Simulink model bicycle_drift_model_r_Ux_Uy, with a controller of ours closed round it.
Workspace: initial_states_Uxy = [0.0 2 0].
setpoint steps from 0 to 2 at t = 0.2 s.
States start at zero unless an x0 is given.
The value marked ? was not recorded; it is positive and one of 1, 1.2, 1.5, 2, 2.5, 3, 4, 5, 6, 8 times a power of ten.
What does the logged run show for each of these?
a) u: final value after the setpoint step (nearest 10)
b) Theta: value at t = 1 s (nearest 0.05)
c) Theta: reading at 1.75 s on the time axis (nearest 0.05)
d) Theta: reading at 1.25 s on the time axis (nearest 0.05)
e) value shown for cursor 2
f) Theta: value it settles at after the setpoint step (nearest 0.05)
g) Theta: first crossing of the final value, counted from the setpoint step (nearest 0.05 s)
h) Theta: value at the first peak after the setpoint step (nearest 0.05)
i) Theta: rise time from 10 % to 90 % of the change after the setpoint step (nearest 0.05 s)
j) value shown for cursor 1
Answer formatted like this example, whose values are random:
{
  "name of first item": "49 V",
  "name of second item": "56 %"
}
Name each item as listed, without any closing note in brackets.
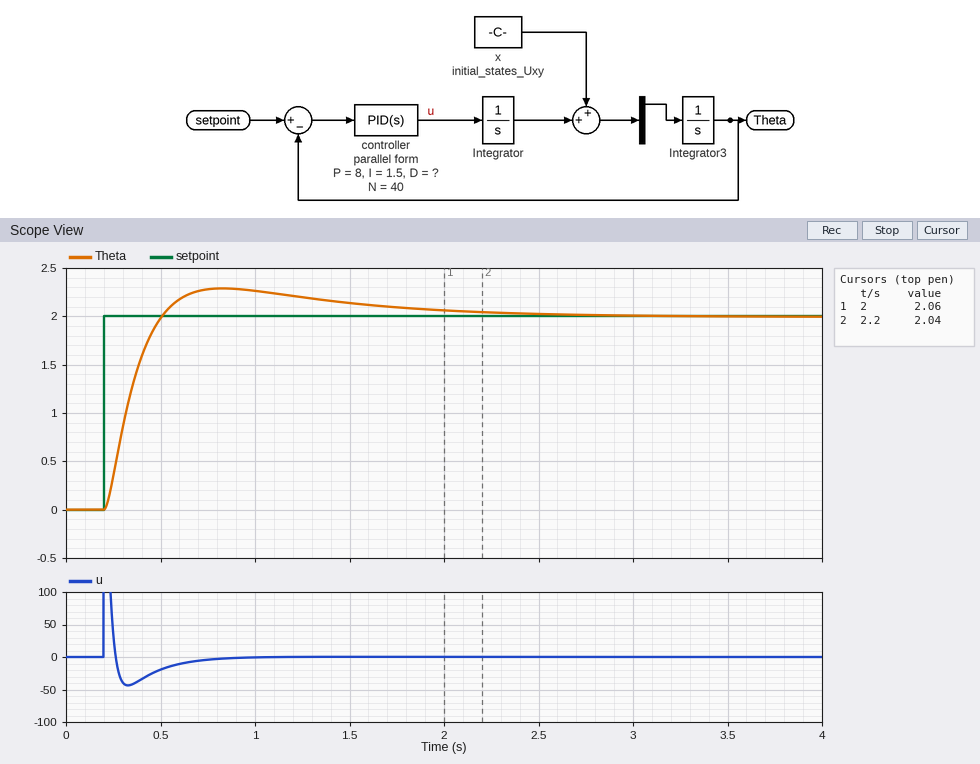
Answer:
{
  "u: final value after the setpoint step": "0",
  "Theta: value at t = 1 s": "2.25",
  "Theta: reading at 1.75 s on the time axis": "2.10",
  "Theta: reading at 1.25 s on the time axis": "2.20",
  "value shown for cursor 2": "2.04",
  "Theta: value it settles at after the setpoint step": "2.00",
  "Theta: first crossing of the final value, counted from the setpoint step": "0.30 s",
  "Theta: value at the first peak after the setpoint step": "2.30",
  "Theta: rise time from 10 % to 90 % of the change after the setpoint step": "0.20 s",
  "value shown for cursor 1": "2.06"
}
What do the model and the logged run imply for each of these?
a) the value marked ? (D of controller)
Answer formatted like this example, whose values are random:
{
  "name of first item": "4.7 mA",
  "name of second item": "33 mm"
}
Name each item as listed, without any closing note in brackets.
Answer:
{
  "the value marked ?": "6"
}
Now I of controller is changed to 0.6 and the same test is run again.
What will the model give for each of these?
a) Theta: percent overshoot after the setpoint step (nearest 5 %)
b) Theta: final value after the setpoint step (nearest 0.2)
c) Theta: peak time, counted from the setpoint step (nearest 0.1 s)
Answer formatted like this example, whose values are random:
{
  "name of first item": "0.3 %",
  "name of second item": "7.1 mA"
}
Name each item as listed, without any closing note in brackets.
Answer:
{
  "Theta: percent overshoot after the setpoint step": "15 %",
  "Theta: final value after the setpoint step": "2.0",
  "Theta: peak time, counted from the setpoint step": "0.6 s"
}
